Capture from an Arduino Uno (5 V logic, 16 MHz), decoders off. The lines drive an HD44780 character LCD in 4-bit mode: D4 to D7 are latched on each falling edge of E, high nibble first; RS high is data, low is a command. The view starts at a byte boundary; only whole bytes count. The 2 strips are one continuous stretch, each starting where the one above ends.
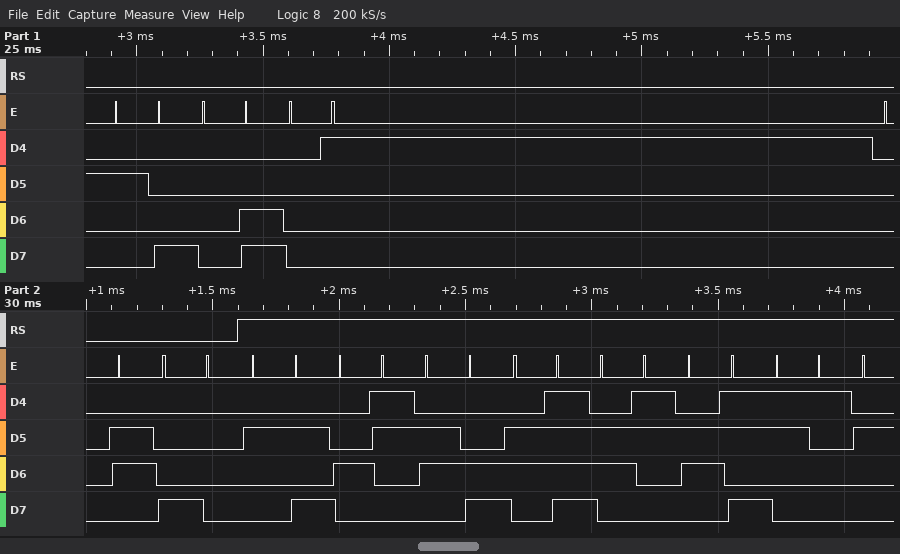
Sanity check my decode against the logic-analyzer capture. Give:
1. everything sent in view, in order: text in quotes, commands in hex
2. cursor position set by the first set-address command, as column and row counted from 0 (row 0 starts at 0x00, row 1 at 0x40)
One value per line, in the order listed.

0x28 0x0C 0x01 0x06 0x80 "*Clock1"
column 0, row 0
